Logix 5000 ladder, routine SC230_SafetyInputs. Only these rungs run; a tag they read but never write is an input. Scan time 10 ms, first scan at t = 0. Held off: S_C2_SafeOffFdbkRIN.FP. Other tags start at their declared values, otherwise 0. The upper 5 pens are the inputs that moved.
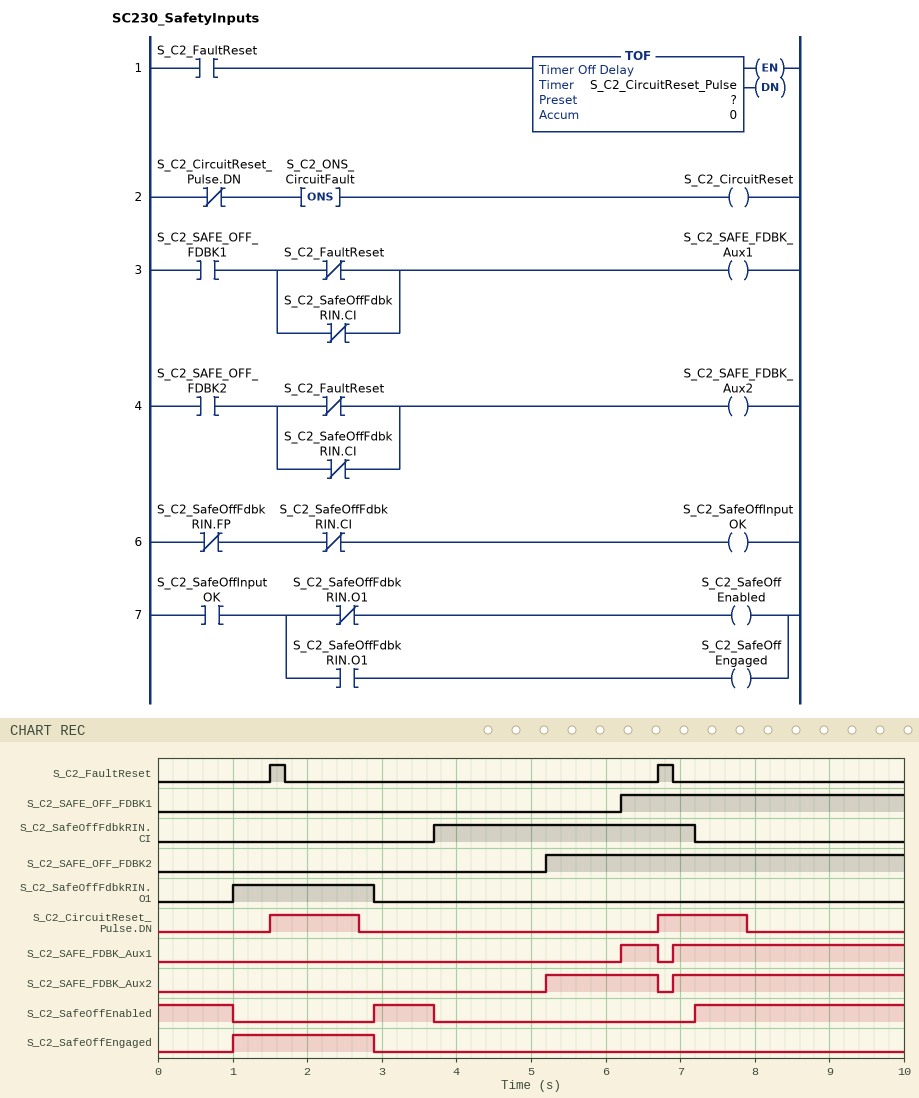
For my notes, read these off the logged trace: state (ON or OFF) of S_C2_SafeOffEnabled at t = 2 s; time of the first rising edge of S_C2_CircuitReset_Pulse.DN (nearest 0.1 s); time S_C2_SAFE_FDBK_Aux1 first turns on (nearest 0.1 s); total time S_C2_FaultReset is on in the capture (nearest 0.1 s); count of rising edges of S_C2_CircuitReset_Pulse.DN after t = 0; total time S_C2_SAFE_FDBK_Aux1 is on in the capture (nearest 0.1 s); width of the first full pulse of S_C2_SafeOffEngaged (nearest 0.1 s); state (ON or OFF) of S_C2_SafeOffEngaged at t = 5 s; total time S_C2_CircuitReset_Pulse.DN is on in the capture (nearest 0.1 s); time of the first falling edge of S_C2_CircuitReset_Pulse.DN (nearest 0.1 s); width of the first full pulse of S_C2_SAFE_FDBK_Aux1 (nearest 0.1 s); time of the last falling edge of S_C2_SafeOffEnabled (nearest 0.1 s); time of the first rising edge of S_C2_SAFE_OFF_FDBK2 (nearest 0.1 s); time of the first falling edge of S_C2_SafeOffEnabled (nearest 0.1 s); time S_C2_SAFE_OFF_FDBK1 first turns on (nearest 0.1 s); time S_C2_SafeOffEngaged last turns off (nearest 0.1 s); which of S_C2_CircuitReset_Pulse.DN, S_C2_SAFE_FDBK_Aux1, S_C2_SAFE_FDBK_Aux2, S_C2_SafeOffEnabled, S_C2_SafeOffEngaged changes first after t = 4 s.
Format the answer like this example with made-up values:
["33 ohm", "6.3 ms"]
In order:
["OFF", "1.5 s", "6.2 s", "0.4 s", "2", "3.6 s", "1.9 s", "OFF", "2.4 s", "2.7 s", "0.5 s", "3.7 s", "5.2 s", "1.0 s", "6.2 s", "2.9 s", "S_C2_SAFE_FDBK_Aux2"]
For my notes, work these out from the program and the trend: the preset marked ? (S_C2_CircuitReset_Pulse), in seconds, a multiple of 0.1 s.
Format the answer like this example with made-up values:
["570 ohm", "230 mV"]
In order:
["1.0 s"]
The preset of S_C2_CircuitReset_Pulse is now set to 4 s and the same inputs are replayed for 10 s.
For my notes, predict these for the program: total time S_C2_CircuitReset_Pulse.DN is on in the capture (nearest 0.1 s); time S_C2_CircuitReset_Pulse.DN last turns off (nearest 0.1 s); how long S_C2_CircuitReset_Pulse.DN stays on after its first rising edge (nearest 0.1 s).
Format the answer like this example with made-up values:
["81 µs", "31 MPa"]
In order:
["7.5 s", "5.7 s", "4.2 s"]
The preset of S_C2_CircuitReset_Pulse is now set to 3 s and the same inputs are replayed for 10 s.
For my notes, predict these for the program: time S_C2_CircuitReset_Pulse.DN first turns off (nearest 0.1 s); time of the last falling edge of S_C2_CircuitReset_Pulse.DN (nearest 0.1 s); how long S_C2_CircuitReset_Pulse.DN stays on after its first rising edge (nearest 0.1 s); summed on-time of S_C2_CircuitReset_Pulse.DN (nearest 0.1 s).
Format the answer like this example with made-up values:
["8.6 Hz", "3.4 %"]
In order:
["4.7 s", "9.9 s", "3.2 s", "6.4 s"]
